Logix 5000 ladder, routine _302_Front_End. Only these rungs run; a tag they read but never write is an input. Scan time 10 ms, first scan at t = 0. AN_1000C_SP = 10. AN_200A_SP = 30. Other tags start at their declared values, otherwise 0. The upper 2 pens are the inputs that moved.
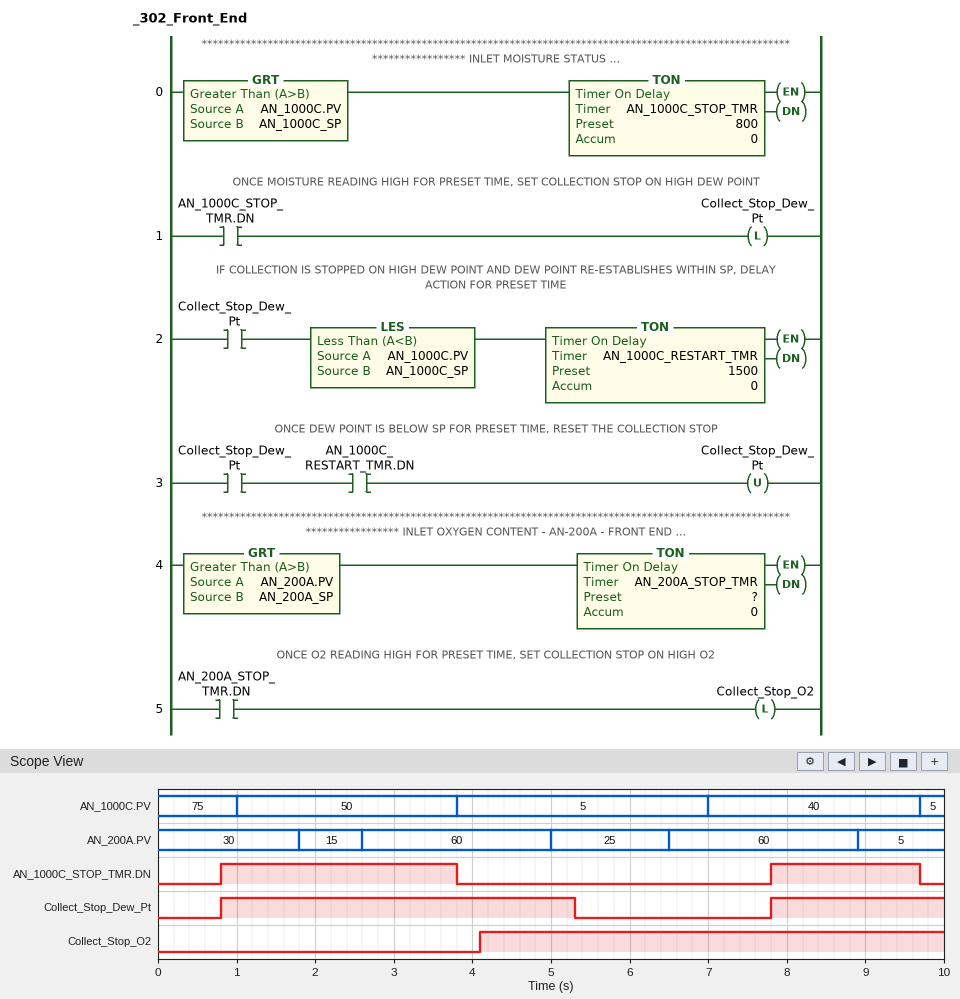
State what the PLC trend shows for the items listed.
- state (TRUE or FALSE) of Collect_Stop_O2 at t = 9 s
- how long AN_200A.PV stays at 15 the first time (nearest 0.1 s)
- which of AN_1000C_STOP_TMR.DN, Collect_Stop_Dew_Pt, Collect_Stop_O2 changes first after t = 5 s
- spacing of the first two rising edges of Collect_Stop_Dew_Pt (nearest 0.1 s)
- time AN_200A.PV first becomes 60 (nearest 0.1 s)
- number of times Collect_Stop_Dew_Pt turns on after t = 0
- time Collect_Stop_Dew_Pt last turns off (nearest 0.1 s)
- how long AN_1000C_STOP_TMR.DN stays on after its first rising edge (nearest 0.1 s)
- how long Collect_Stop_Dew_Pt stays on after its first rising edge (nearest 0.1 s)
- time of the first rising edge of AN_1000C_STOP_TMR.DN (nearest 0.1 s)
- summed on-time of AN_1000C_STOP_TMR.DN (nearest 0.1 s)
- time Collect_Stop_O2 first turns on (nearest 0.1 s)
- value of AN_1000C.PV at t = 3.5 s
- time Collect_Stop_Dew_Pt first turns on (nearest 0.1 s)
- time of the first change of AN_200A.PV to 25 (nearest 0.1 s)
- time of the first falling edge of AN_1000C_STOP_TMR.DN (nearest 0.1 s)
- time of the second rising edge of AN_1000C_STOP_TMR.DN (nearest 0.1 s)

TRUE
0.8 s
Collect_Stop_Dew_Pt
7.0 s
2.6 s
2
5.3 s
3.0 s
4.5 s
0.8 s
4.9 s
4.1 s
50
0.8 s
5.0 s
3.8 s
7.8 s
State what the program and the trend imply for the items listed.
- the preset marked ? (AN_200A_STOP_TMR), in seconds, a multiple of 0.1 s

1.5 s
